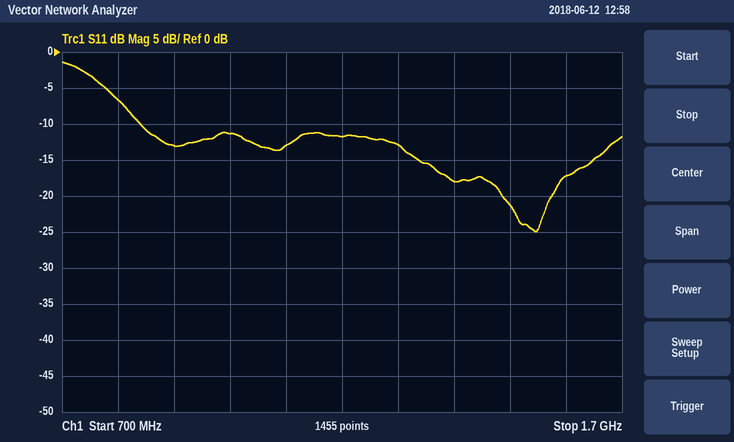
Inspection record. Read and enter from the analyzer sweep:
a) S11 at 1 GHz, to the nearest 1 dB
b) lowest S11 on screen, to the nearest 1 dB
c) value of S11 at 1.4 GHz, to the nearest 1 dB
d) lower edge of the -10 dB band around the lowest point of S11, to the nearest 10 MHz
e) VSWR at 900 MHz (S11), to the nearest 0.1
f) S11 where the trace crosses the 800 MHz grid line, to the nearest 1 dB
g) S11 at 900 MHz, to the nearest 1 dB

-11 dB
-25 dB
-18 dB
840 MHz
1.6
-7 dB
-13 dB
